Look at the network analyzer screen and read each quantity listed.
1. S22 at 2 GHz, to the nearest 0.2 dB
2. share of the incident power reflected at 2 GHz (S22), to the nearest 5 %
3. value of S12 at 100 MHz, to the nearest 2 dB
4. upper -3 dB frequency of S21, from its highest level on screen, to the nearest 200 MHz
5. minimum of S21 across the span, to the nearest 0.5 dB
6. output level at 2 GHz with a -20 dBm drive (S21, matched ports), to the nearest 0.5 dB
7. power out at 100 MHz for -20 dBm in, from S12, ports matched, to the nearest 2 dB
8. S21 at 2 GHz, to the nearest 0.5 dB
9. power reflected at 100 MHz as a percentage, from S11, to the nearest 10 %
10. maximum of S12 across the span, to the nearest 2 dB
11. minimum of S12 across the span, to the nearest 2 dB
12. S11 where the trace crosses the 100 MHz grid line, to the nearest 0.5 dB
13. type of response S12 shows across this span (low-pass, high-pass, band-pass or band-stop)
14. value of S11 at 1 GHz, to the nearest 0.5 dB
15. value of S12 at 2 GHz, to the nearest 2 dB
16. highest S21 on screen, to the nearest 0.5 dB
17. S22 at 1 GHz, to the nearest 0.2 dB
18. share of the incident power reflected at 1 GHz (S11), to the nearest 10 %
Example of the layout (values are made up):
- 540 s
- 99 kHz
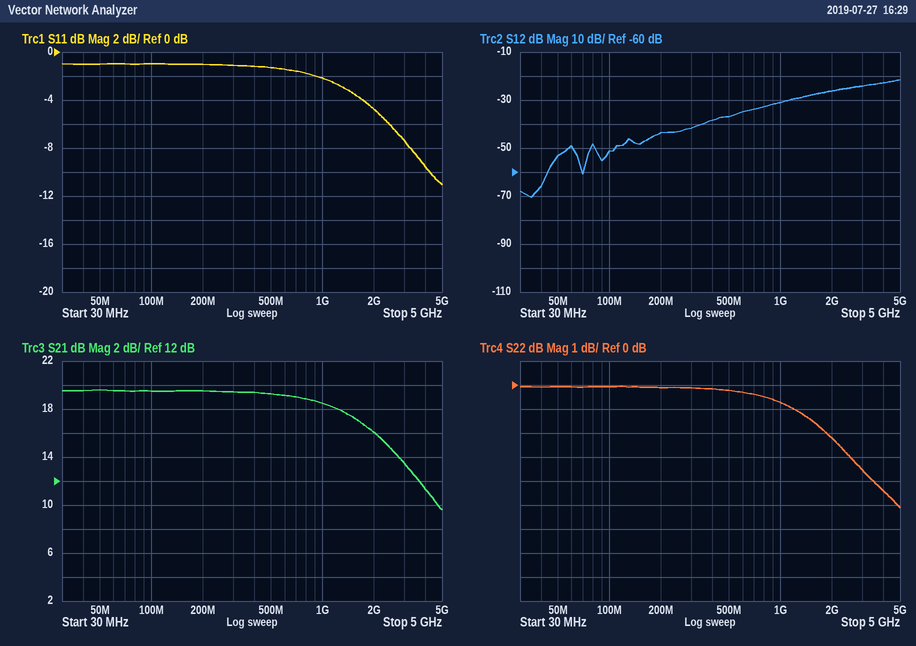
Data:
- -2.2 dB
- 60 %
- -52 dB
- 1.8 GHz
- 9.5 dB
- -4.0 dBm
- -72 dBm
- 16.0 dB
- 80 %
- -22 dB
- -70 dB
- -1.0 dB
- high-pass
- -2.0 dB
- -26 dB
- 19.5 dB
- -0.8 dB
- 60 %
